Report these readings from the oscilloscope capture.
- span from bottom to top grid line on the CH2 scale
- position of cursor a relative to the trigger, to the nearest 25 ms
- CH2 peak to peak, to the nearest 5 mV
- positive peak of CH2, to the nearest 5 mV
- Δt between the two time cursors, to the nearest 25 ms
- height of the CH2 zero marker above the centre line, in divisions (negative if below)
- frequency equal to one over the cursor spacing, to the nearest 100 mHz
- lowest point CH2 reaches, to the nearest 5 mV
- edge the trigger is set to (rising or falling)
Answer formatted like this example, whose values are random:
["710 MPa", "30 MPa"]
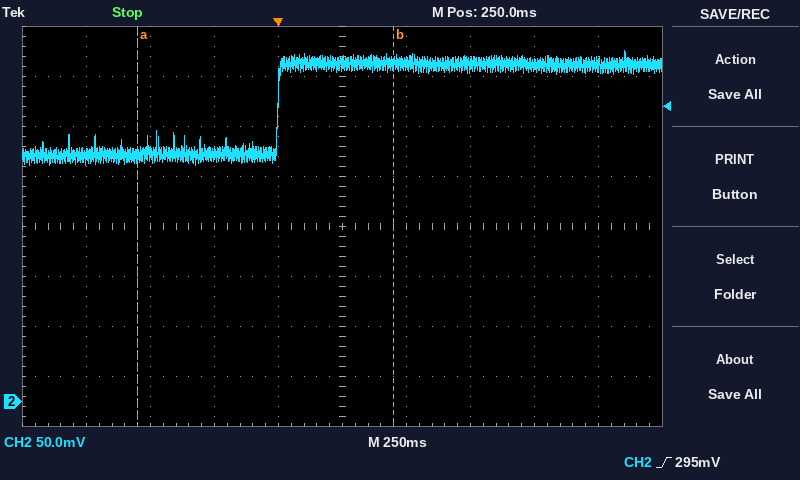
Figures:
["400 mV", "-550 ms", "115 mV", "350 mV", "1.000 s", "-3.5 div", "1.0 Hz", "235 mV", "rising"]
